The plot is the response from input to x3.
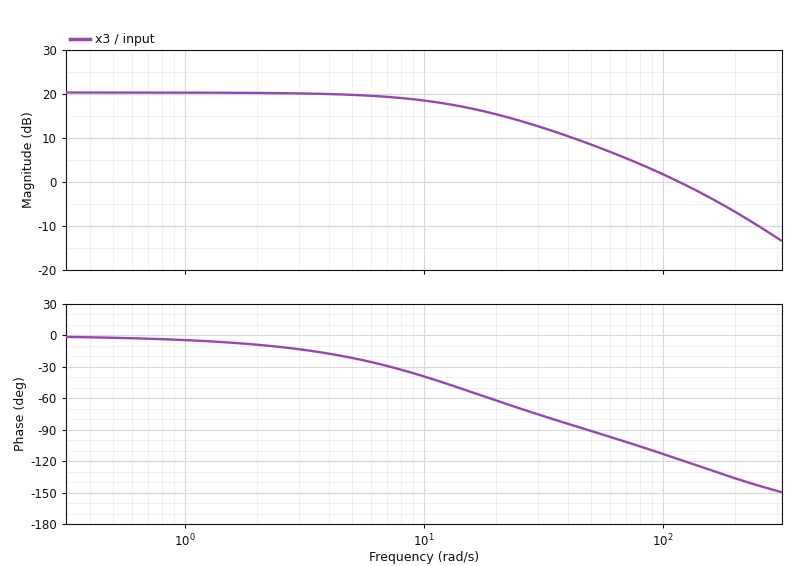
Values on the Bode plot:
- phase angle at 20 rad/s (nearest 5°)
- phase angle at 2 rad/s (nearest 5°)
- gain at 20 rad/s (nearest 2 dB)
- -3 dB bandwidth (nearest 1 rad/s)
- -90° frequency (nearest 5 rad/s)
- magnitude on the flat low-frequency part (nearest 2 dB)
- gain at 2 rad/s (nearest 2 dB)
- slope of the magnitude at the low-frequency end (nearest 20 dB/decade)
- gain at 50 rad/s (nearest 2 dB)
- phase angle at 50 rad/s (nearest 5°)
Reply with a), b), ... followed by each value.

a) -60°
b) -10°
c) 16 dB
d) 14 rad/s
e) 50 rad/s
f) 20 dB
g) 20 dB
h) 0 dB/decade
i) 8 dB
j) -90°
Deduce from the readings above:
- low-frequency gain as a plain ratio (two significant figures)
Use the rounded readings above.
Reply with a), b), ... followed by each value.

a) 10
